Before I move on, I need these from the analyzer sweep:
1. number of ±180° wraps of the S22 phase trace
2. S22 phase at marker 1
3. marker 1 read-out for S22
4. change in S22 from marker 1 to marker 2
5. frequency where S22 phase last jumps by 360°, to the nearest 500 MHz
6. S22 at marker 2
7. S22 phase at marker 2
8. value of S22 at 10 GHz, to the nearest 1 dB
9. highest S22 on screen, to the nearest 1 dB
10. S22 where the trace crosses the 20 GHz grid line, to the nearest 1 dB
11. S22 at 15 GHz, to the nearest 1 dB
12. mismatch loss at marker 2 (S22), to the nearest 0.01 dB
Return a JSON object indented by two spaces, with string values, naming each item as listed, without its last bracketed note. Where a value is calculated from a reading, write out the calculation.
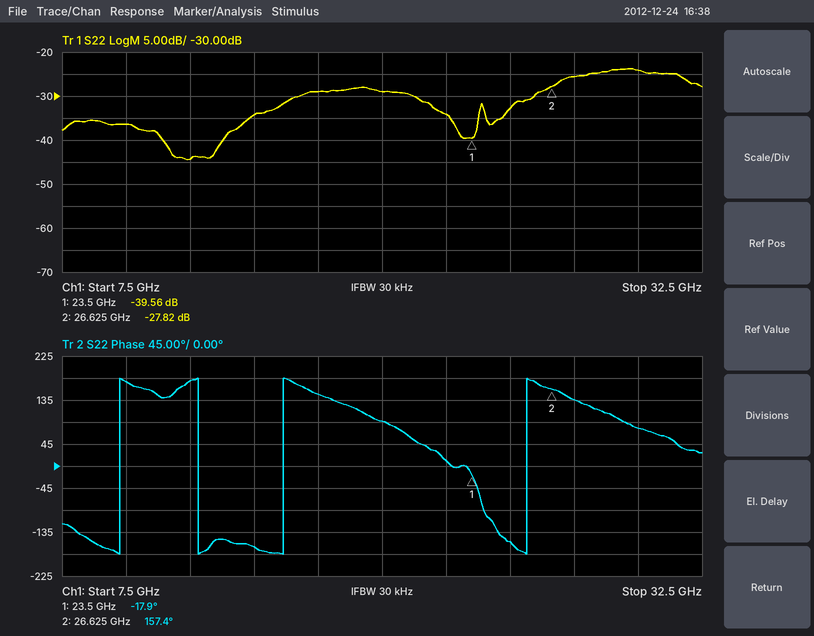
{
  "number of ±180° wraps of the S22 phase trace": "4",
  "S22 phase at marker 1": "-17.9°",
  "marker 1 read-out for S22": "-39.56 dB",
  "change in S22 from marker 1 to marker 2": "-27.82 − (-39.56) = 11.74 dB",
  "frequency where S22 phase last jumps by 360°, to the nearest 500 MHz": "25.5 GHz",
  "S22 at marker 2": "-27.82 dB",
  "S22 phase at marker 2": "157.4°",
  "value of S22 at 10 GHz, to the nearest 1 dB": "-36 dB",
  "highest S22 on screen, to the nearest 1 dB": "-24 dB",
  "S22 where the trace crosses the 20 GHz grid line, to the nearest 1 dB": "-29 dB",
  "S22 at 15 GHz, to the nearest 1 dB": "-34 dB",
  "mismatch loss at marker 2 (S22), to the nearest 0.01 dB": "−10 log10(1 − 10^(-27.82/10)) ≈ 0.01 dB"
}
